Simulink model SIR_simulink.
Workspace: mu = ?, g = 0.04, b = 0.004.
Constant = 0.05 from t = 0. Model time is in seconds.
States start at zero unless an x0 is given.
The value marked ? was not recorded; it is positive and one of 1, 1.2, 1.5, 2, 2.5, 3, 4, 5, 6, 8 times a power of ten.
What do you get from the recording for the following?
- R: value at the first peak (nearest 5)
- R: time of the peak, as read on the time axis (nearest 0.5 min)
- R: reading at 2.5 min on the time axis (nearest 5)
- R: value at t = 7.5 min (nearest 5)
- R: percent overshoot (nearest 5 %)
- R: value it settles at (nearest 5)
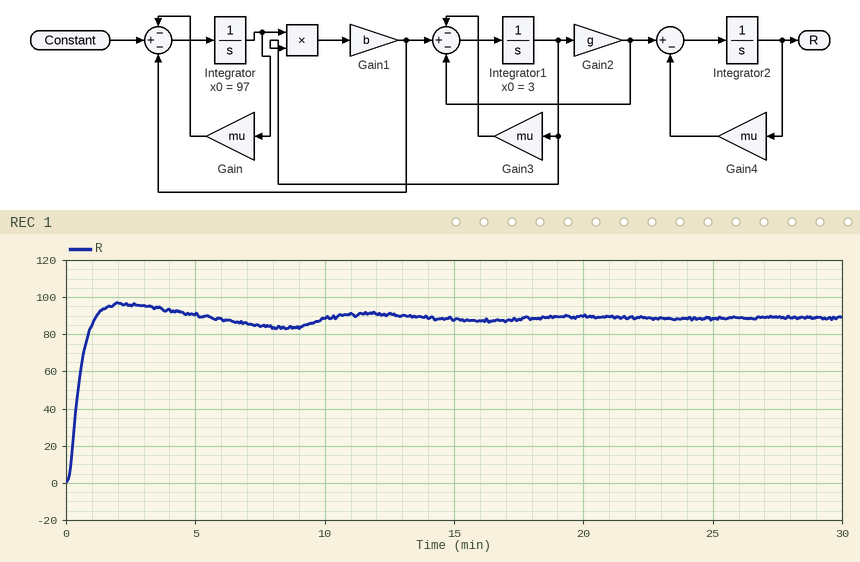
95
2.0 min
95
85
10 %
90
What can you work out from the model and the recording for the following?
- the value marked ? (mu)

0.0005
